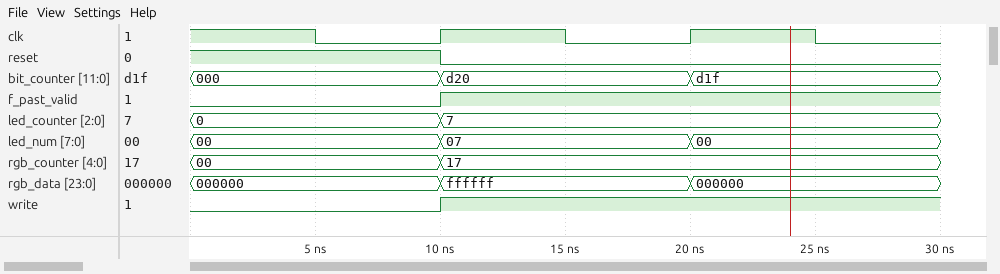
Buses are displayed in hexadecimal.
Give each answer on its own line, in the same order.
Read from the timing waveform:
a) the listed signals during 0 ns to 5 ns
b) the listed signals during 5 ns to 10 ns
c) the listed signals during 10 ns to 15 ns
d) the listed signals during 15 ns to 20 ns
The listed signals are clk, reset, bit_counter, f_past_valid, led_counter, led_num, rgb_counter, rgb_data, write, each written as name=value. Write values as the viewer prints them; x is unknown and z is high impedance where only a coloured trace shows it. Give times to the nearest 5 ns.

clk=1, reset=1, bit_counter=000, f_past_valid=0, led_counter=0, led_num=00, rgb_counter=00, rgb_data=000000, write=0
clk=0, reset=1, bit_counter=000, f_past_valid=0, led_counter=0, led_num=00, rgb_counter=00, rgb_data=000000, write=0
clk=1, reset=0, bit_counter=d20, f_past_valid=1, led_counter=7, led_num=07, rgb_counter=17, rgb_data=ffffff, write=1
clk=0, reset=0, bit_counter=d20, f_past_valid=1, led_counter=7, led_num=07, rgb_counter=17, rgb_data=ffffff, write=1
